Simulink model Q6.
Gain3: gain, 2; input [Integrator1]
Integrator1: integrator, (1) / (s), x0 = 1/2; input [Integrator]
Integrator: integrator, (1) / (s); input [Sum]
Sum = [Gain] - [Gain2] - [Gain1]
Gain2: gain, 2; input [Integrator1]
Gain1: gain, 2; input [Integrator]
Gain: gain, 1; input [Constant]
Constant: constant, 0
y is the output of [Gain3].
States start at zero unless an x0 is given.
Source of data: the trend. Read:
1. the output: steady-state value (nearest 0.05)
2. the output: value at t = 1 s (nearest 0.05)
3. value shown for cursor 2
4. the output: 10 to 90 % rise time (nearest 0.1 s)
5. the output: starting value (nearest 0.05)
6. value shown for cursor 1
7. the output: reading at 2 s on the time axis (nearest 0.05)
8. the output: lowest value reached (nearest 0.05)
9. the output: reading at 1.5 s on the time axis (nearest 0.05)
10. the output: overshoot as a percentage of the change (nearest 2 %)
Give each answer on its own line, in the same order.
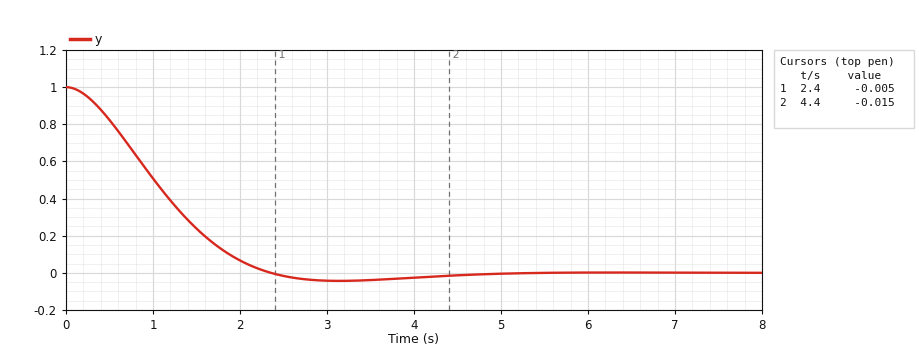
0.00
0.50
-0.015
1.5 s
1.00
-0.005
0.05
-0.05
0.25
4 %
